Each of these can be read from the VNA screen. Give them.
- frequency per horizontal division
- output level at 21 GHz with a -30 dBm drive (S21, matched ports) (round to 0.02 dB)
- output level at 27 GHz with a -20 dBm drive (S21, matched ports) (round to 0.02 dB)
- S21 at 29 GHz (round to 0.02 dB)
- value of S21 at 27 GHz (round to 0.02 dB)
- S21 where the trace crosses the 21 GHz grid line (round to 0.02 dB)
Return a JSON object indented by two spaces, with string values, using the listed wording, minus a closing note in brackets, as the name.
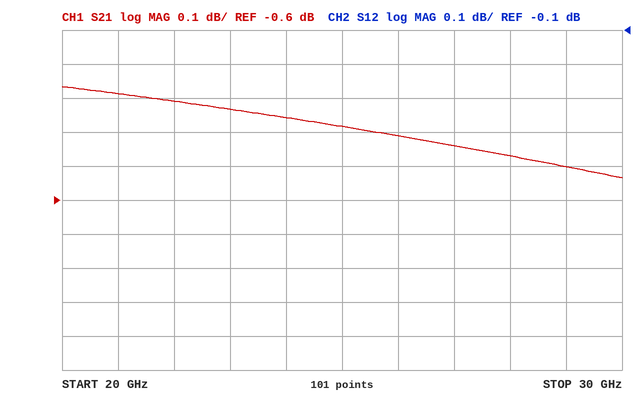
{
  "frequency per horizontal division": "1 GHz",
  "output level at 21 GHz with a -30 dBm drive (S21, matched ports)": "-30.28 dBm",
  "output level at 27 GHz with a -20 dBm drive (S21, matched ports)": "-20.44 dBm",
  "S21 at 29 GHz": "-0.50 dB",
  "value of S21 at 27 GHz": "-0.44 dB",
  "S21 where the trace crosses the 21 GHz grid line": "-0.28 dB"
}
